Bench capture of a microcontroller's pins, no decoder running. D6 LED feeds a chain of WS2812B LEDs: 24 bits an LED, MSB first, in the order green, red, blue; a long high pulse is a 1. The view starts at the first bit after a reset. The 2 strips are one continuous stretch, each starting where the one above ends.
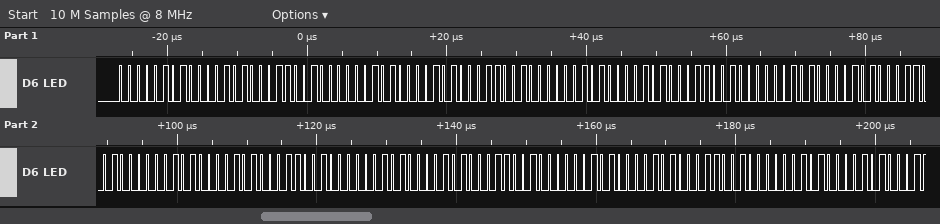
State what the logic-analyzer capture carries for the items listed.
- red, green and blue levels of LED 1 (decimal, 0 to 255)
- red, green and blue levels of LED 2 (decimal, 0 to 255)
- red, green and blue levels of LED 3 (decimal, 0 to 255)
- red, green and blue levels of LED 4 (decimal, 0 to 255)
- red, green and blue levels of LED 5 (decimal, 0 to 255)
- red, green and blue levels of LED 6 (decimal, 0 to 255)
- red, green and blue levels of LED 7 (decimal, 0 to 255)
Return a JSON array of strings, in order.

["10, 5, 50", "10, 5, 50", "10, 5, 50", "10, 5, 50", "10, 5, 50", "10, 5, 50", "10, 5, 50"]
